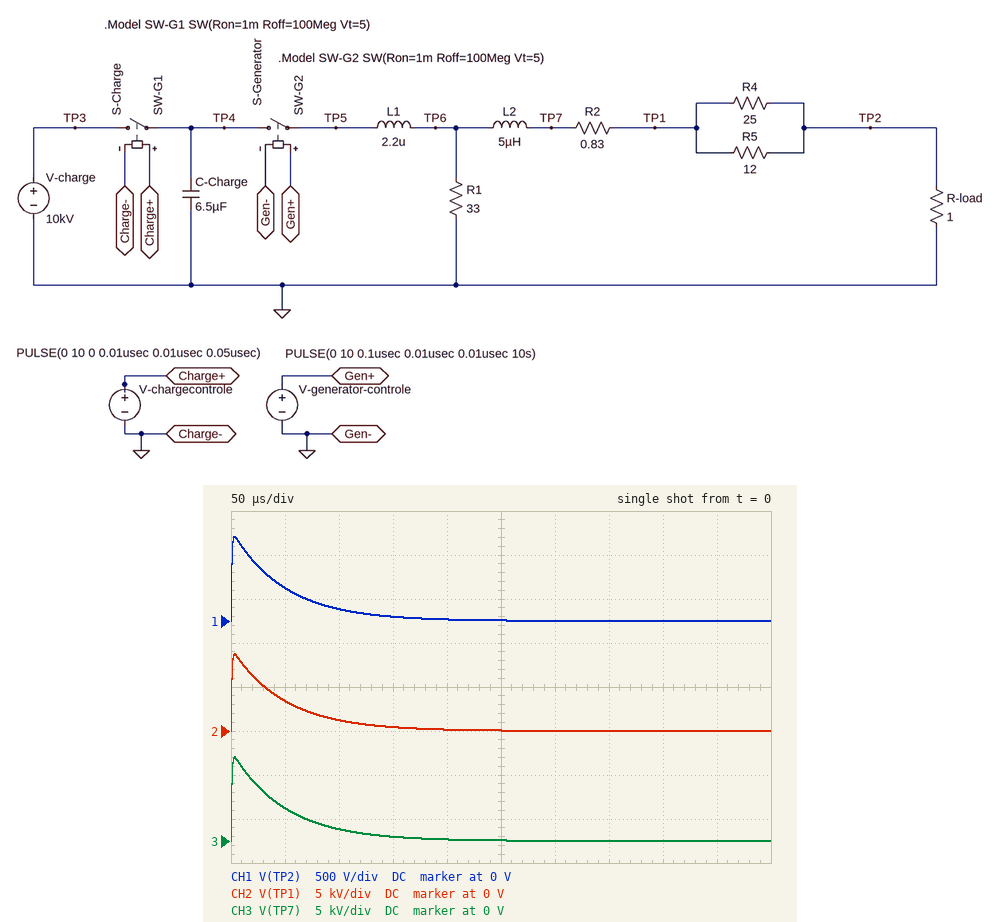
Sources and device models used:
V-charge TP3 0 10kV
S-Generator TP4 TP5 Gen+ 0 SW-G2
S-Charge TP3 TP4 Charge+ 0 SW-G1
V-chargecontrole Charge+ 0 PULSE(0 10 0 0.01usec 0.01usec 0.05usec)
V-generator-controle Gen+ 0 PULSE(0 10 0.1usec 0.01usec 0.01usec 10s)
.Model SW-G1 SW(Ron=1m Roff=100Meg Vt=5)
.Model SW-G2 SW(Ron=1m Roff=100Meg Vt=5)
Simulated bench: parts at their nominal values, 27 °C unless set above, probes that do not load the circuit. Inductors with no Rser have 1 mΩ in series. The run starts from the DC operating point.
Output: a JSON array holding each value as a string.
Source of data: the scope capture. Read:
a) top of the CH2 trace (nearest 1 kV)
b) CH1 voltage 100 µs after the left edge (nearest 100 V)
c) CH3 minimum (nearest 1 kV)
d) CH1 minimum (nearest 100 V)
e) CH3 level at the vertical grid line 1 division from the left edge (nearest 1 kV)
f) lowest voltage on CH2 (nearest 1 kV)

["9 kV", "100 V", "0 V", "0 V", "4 kV", "0 V"]
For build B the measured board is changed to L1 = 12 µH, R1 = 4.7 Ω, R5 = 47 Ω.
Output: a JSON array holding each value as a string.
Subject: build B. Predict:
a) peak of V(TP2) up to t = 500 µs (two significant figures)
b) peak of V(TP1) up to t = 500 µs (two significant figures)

["440 V", "7.7 kV"]
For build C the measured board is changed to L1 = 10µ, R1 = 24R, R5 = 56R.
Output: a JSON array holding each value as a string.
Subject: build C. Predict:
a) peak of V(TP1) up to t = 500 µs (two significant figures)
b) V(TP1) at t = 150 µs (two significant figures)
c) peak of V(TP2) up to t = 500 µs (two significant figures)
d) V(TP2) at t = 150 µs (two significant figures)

["9.1 kV", "1.1 kV", "500 V", "60 V"]
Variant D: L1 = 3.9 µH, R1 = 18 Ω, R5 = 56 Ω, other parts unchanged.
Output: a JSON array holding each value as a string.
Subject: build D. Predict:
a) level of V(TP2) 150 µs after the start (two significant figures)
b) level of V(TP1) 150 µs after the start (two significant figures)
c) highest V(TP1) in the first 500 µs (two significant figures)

["43 V", "790 V", "9.2 kV"]
